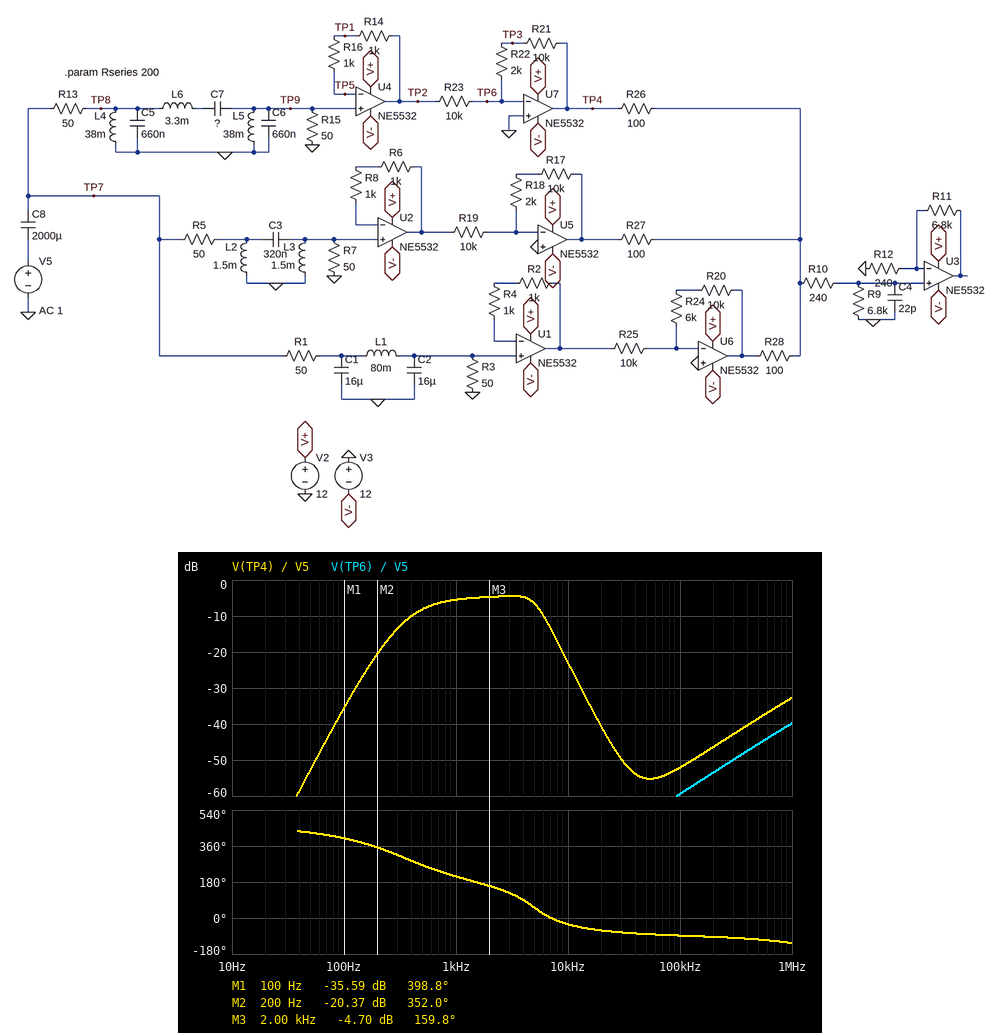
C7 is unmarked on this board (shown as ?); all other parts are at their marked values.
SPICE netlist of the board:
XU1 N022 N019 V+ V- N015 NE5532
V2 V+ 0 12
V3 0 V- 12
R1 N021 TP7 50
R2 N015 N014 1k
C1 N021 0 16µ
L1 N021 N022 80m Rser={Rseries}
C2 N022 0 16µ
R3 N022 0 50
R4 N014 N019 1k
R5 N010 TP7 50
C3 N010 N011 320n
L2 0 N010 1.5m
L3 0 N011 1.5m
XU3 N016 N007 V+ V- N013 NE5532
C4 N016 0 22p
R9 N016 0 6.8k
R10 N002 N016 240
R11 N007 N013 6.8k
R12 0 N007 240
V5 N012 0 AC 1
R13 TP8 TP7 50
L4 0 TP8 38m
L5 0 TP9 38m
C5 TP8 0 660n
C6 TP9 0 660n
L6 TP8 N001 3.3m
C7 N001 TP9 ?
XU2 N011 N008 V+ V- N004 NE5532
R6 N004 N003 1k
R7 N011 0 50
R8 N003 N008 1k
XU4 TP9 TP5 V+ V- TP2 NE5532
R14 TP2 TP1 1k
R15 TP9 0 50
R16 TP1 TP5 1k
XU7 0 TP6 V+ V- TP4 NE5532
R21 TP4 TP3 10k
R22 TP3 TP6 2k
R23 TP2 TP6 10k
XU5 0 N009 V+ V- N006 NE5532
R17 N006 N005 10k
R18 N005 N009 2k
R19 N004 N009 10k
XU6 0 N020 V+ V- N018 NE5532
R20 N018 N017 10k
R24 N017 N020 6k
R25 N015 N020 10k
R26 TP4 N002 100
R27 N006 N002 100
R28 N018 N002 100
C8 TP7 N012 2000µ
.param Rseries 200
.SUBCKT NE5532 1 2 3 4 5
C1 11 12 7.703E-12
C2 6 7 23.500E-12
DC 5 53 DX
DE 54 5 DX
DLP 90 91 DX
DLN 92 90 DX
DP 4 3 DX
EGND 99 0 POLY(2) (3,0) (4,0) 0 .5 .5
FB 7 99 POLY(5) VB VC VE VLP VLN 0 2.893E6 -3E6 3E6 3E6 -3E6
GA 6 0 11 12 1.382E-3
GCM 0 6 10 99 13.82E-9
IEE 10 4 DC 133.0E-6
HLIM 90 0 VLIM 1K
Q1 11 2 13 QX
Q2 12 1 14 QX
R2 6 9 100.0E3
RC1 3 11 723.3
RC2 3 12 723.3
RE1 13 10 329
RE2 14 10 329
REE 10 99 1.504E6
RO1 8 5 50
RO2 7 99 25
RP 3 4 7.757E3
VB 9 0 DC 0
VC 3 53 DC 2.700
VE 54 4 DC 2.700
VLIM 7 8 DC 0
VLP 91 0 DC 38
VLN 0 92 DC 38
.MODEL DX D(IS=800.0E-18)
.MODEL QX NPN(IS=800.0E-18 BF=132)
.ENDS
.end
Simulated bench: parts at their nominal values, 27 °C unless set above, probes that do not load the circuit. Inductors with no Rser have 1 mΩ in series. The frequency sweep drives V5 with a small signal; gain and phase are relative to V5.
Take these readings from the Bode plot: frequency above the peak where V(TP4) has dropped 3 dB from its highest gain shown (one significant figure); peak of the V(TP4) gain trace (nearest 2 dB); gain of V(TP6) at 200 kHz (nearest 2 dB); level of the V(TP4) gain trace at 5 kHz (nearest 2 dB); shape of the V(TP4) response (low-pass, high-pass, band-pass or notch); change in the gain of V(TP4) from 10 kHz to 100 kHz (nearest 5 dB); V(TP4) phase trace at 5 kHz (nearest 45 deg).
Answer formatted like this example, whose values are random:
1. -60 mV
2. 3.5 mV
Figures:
1. 5 kHz
2. -4 dB
3. -54 dB
4. -6 dB
5. band-pass
6. -30 dB
7. 45 deg
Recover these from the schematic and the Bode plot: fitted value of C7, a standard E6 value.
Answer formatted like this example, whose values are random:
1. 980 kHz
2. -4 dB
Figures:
1. 2.2 µF
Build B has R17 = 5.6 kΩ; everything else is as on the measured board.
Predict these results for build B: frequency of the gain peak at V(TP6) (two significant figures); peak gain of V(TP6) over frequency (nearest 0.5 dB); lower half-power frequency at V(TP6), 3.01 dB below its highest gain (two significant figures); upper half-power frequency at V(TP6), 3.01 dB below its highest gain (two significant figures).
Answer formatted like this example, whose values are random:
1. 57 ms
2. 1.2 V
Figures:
1. 4.7 MHz
2. -35.0 dB
3. 2.1 MHz
4. 8.4 MHz
